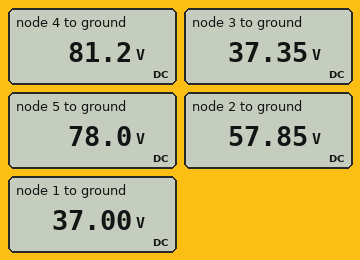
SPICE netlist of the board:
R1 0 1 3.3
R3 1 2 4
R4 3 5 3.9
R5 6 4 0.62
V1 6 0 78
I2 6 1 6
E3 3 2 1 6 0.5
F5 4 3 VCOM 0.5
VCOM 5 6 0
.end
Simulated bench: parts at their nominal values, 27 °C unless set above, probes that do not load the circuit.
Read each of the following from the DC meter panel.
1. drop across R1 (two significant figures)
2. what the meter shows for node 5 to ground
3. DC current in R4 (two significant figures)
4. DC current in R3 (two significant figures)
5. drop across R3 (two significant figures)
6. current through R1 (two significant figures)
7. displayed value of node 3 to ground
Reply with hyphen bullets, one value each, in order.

- 37 V
- 78.0 V
- 10 A
- 5.2 A
- 21 V
- 11 A
- 37.35 V
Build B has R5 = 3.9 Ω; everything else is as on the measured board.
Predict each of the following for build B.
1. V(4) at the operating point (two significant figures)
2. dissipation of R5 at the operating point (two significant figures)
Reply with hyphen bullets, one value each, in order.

- 98 V
- 110 W
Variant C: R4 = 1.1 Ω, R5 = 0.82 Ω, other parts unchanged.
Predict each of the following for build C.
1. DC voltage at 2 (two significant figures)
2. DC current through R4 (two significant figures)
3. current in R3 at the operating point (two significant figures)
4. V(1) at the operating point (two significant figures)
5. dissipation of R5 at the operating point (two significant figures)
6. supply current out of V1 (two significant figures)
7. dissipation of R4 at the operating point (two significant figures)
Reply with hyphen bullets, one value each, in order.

- 77 V
- 16 A
- 7.8 A
- 46 V
- 50 W
- 14 A
- 270 W
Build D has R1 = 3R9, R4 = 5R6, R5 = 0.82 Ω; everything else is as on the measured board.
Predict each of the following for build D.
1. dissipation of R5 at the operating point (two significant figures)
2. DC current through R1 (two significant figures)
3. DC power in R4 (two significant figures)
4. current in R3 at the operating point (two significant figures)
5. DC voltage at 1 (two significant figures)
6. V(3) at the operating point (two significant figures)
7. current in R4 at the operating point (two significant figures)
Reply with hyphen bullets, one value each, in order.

- 12 W
- 9.9 A
- 340 W
- 3.9 A
- 39 V
- 34 V
- 7.8 A
